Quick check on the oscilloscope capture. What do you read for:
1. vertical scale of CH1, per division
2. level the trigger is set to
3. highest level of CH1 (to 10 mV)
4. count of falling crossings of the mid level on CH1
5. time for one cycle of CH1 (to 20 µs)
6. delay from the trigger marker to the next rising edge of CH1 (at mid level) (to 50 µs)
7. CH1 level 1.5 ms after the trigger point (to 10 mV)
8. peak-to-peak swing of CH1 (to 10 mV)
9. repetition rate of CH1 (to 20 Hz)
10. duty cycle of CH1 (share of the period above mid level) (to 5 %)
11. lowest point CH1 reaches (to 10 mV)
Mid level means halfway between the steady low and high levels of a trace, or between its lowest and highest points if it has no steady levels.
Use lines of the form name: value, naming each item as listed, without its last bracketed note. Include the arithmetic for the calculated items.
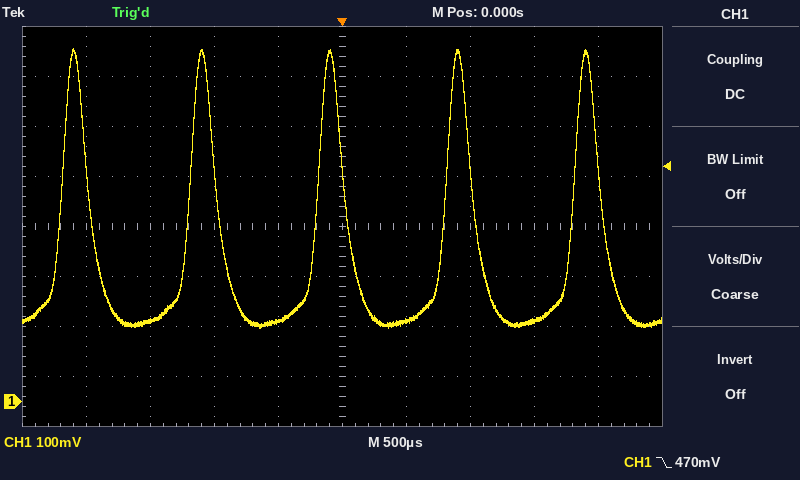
vertical scale of CH1, per division: 100 mV
level the trigger is set to: 470 mV
highest level of CH1: 710 mV
count of falling crossings of the mid level on CH1: 5
time for one cycle of CH1: 1.00 ms
delay from the trigger marker to the next rising edge of CH1 (at mid level): 800 µs
CH1 level 1.5 ms after the trigger point: 160 mV
peak-to-peak swing of CH1: 710 mV − (150 mV) = 560 mV
repetition rate of CH1: 1 / 1.00 ms ≈ 1.00 kHz
duty cycle of CH1 (share of the period above mid level): 20 %
lowest point CH1 reaches: 150 mV
